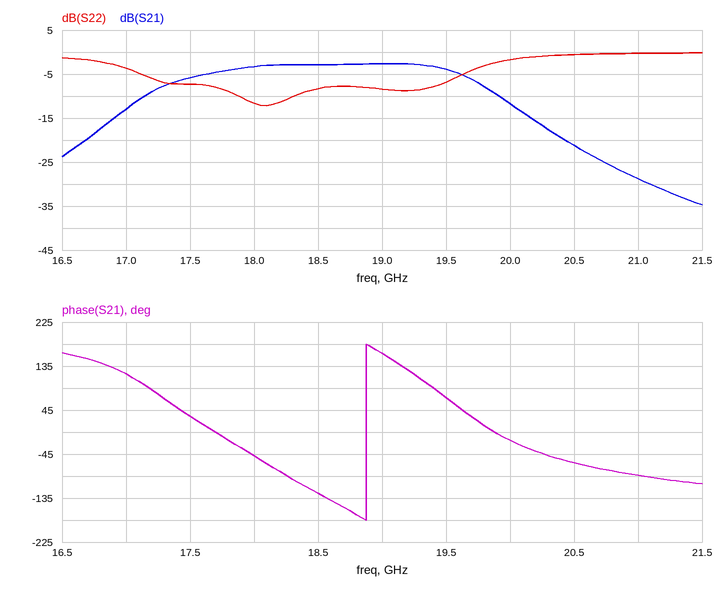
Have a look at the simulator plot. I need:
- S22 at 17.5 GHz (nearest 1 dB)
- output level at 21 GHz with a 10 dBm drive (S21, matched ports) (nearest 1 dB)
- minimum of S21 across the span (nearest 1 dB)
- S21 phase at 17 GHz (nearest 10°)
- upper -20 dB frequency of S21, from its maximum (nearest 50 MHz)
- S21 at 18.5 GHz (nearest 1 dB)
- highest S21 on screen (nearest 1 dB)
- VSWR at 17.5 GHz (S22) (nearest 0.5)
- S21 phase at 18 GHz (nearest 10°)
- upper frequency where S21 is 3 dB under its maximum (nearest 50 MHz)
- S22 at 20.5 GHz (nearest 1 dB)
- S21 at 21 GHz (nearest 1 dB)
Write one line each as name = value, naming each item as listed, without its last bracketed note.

S22 at 17.5 GHz = -7 dB
output level at 21 GHz with a 10 dBm drive (S21, matched ports) = -19 dBm
minimum of S21 across the span = -35 dB
S21 phase at 17 GHz = 120°
upper -20 dB frequency of S21, from its maximum = 20.60 GHz
S21 at 18.5 GHz = -3 dB
highest S21 on screen = -3 dB
VSWR at 17.5 GHz (S22) = 2.5
S21 phase at 18 GHz = -50°
upper frequency where S21 is 3 dB under its maximum = 19.65 GHz
S22 at 20.5 GHz = -1 dB
S21 at 21 GHz = -29 dB
